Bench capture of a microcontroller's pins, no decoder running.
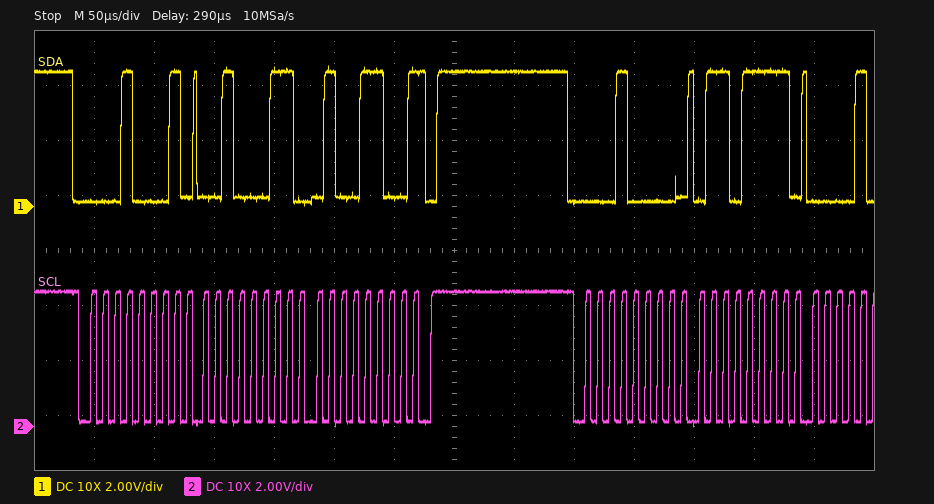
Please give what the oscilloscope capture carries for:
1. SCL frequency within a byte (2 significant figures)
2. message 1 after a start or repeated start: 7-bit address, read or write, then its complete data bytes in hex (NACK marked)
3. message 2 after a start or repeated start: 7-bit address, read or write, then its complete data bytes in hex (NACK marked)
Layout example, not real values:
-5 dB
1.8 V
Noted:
100 kHz
0x08 read: 23 4C NACK
0x08 write: 6F
